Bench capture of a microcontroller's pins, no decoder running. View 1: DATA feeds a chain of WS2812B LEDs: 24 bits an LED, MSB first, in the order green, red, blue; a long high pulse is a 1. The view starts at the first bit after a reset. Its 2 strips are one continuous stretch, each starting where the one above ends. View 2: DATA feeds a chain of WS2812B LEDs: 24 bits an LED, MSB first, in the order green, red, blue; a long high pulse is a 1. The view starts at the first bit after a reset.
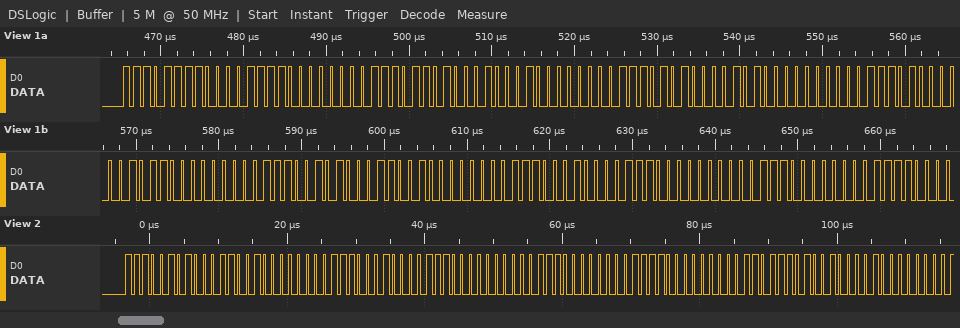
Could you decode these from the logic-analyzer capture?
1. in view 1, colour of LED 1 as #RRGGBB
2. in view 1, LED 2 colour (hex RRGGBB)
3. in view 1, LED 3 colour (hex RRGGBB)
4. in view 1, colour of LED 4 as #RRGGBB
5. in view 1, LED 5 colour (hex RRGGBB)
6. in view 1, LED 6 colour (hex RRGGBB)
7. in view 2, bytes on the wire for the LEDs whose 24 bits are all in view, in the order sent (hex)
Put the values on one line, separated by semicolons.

#0FEF00; #11ED00; #14EA00; #16E800; #19E500; #1CE200; E5 19 00 E2 1C 00 E0 1E 00 DD 21 00
